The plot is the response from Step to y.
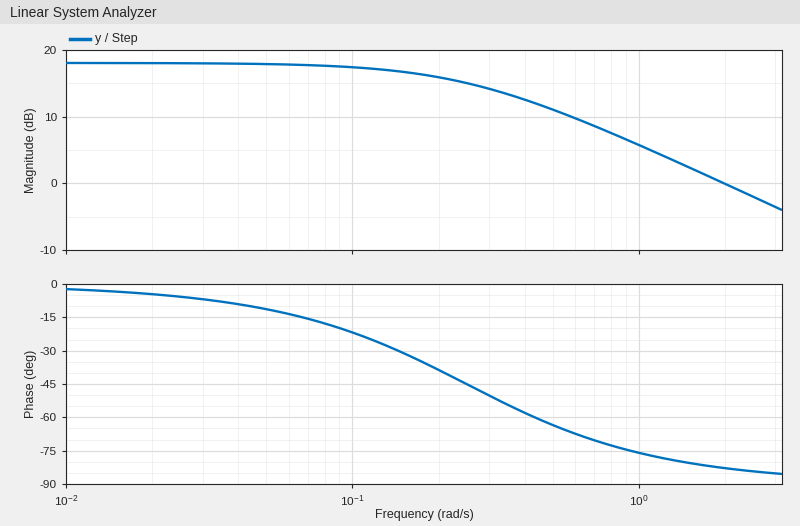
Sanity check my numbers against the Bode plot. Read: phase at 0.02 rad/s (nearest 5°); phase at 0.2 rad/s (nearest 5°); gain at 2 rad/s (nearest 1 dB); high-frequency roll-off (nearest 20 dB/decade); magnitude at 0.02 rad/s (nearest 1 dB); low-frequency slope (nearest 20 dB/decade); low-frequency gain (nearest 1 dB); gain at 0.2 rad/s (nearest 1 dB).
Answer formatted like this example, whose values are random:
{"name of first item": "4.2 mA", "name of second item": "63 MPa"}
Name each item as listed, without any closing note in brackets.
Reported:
{"phase at 0.02 rad/s": "-5°", "phase at 0.2 rad/s": "-40°", "gain at 2 rad/s": "0 dB", "high-frequency roll-off": "-20 dB/decade", "magnitude at 0.02 rad/s": "18 dB", "low-frequency slope": "0 dB/decade", "low-frequency gain": "18 dB", "gain at 0.2 rad/s": "16 dB"}
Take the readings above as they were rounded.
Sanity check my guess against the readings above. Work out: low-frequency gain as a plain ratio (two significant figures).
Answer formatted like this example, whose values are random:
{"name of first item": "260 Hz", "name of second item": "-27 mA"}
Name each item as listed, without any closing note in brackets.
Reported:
{"low-frequency gain as a plain ratio": "7.9"}
